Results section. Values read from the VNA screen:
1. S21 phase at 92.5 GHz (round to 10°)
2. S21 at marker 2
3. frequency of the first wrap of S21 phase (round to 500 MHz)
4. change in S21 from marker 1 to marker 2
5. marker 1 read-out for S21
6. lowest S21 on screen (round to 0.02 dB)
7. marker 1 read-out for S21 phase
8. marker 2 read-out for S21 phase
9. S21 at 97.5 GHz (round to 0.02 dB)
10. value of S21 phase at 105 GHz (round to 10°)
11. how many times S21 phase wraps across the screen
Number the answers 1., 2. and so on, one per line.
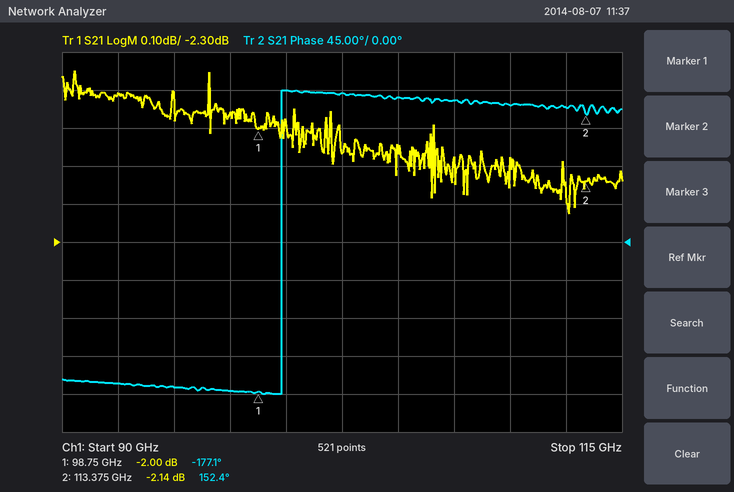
1. -170°
2. -2.14 dB
3. 100.0 GHz
4. -0.14 dB
5. -2.00 dB
6. -2.22 dB
7. -177.1°
8. 152.4°
9. -1.96 dB
10. 170°
11. 1
